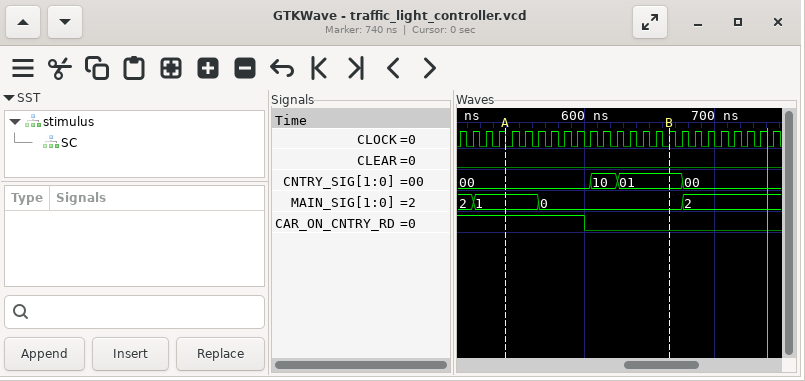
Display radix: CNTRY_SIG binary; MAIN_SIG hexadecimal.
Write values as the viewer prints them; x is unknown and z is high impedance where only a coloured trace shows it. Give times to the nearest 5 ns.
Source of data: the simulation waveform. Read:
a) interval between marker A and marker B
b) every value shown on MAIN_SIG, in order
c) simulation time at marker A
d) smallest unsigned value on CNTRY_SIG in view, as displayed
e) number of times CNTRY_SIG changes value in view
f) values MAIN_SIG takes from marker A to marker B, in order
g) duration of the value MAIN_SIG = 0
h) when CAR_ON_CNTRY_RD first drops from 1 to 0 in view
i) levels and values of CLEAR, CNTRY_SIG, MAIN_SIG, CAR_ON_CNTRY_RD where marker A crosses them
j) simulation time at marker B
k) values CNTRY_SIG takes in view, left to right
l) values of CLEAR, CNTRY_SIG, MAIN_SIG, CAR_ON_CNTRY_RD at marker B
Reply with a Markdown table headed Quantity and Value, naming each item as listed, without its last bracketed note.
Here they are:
| Quantity | Value |
|---|---|
| interval between marker A and marker B | 125 ns |
| every value shown on MAIN_SIG, in order | 2, 1, 0, 2 |
| simulation time at marker A | 540 ns |
| smallest unsigned value on CNTRY_SIG in view, as displayed | 00 |
| number of times CNTRY_SIG changes value in view | 3 |
| values MAIN_SIG takes from marker A to marker B, in order | 1, 0 |
| duration of the value MAIN_SIG = 0 | 110 ns |
| when CAR_ON_CNTRY_RD first drops from 1 to 0 in view | 600 ns |
| levels and values of CLEAR, CNTRY_SIG, MAIN_SIG, CAR_ON_CNTRY_RD where marker A crosses them | CLEAR=0, CNTRY_SIG=00, MAIN_SIG=1, CAR_ON_CNTRY_RD=1 |
| simulation time at marker B | 665 ns |
| values CNTRY_SIG takes in view, left to right | 00, 10, 01, 00 |
| values of CLEAR, CNTRY_SIG, MAIN_SIG, CAR_ON_CNTRY_RD at marker B | CLEAR=0, CNTRY_SIG=01, MAIN_SIG=0, CAR_ON_CNTRY_RD=0 |
